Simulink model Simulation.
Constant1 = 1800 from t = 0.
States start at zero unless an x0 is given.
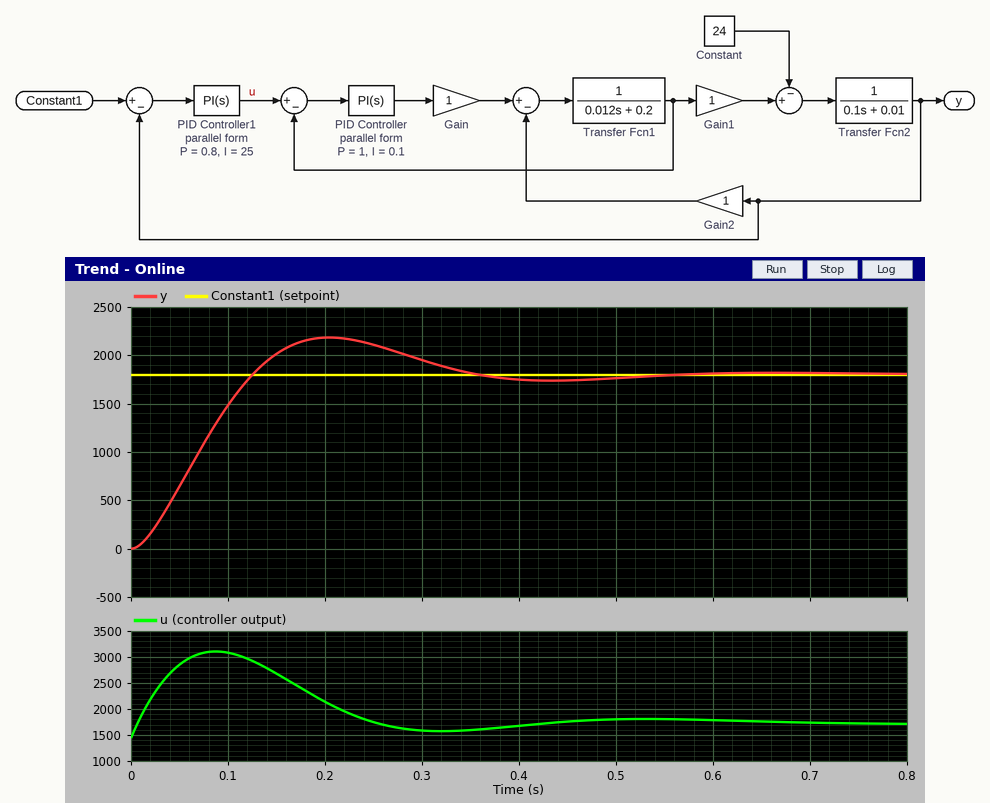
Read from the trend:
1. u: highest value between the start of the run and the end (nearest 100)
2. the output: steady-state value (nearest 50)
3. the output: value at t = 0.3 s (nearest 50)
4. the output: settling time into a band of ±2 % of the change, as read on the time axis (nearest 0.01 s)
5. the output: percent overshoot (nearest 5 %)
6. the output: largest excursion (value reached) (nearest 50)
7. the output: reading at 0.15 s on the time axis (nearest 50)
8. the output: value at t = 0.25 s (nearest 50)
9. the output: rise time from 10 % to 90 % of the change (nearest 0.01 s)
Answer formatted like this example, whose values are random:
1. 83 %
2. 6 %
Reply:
1. 3100
2. 1800
3. 1950
4. 0.51 s
5. 20 %
6. 2200
7. 2000
8. 2100
9. 0.09 s
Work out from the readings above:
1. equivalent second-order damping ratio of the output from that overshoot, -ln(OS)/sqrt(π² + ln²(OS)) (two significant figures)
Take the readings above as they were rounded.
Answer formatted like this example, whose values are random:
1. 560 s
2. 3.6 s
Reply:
1. 0.46
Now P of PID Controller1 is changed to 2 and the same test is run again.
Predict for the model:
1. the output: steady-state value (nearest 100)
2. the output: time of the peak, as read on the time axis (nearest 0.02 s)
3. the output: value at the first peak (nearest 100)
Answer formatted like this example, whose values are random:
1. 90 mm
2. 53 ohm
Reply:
1. 1800
2. 0.18 s
3. 1900
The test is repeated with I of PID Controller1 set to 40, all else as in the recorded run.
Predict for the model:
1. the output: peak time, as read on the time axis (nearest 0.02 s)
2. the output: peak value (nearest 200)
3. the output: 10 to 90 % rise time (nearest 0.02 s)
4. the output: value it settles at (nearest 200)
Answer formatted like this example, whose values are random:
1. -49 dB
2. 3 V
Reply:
1. 0.16 s
2. 2400
3. 0.06 s
4. 1800
